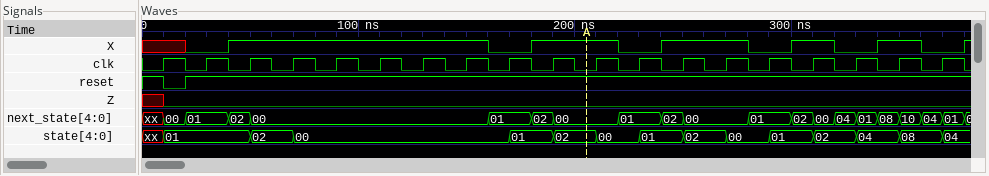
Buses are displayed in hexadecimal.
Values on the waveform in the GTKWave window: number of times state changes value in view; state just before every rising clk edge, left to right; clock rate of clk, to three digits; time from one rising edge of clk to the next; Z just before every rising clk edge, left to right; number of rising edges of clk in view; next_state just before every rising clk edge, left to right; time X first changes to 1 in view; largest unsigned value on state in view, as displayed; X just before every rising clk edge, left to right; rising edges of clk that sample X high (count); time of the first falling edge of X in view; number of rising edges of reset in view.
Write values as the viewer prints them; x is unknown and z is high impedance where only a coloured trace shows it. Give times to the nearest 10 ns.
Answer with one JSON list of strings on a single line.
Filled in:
["14", "xx, 01, 01, 02, 00, 00, 00, 00, 00, 01, 02, 00, 01, 02, 00, 01, 02, 04, 08", "50.0 MHz", "20 ns", "x 0 0 0 0 0 0 0 0 0 0 0 0 0 0 0 0 0 0", "19", "xx, 01, 02, 00, 00, 00, 00, 00, 01, 02, 00, 01, 02, 00, 01, 02, 04, 08, 04", "40 ns", "08", "x 0 1 1 1 1 1 1 0 1 1 0 1 1 0 1 0 1 0", "12", "160 ns", "1"]
